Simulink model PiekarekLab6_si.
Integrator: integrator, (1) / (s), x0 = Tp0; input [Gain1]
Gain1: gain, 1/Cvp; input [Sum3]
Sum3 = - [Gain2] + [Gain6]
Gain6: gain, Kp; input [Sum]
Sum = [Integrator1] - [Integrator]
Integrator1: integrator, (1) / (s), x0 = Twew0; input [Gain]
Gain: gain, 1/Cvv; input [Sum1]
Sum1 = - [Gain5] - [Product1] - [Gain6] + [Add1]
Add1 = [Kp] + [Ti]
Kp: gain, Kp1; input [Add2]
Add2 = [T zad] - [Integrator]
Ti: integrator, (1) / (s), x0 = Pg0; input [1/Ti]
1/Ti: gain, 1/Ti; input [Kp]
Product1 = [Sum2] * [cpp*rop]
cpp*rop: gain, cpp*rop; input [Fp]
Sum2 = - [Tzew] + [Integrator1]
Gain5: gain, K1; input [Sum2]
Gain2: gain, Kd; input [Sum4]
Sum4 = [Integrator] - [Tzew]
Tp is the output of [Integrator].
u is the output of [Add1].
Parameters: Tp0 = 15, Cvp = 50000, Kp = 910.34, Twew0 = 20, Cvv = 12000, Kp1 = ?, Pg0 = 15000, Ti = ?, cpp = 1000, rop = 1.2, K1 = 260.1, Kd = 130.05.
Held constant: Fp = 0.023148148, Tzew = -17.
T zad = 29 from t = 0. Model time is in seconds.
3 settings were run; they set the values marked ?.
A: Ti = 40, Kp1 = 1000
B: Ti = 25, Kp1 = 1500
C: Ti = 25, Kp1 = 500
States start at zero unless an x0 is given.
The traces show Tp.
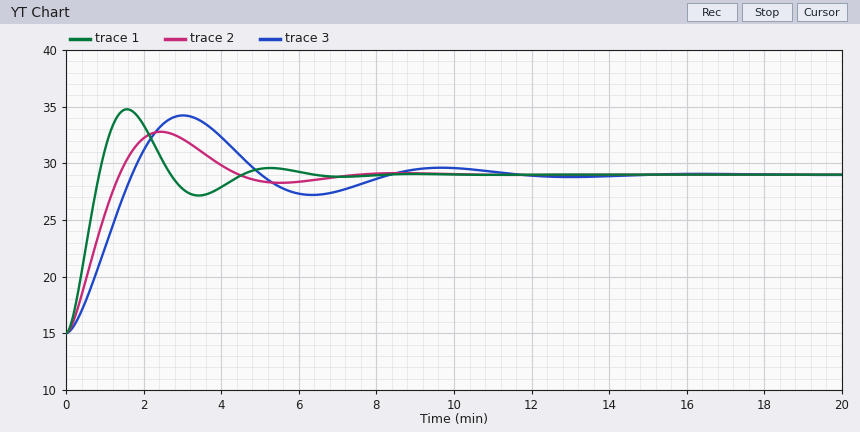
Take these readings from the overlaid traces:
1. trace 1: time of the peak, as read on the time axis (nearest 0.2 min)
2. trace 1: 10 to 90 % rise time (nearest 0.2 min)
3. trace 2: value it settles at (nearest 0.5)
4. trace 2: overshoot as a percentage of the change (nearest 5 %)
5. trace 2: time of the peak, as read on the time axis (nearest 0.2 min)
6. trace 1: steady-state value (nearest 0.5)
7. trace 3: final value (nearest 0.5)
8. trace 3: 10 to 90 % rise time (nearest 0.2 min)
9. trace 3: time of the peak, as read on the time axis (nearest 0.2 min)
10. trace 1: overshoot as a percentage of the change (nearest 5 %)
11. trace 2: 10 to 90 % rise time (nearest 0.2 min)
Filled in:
1.6 min
0.6 min
29.0
25 %
2.4 min
29.0
29.0
1.2 min
3.0 min
40 %
1.0 min
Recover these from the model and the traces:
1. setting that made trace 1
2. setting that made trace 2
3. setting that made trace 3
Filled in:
B
A
C
